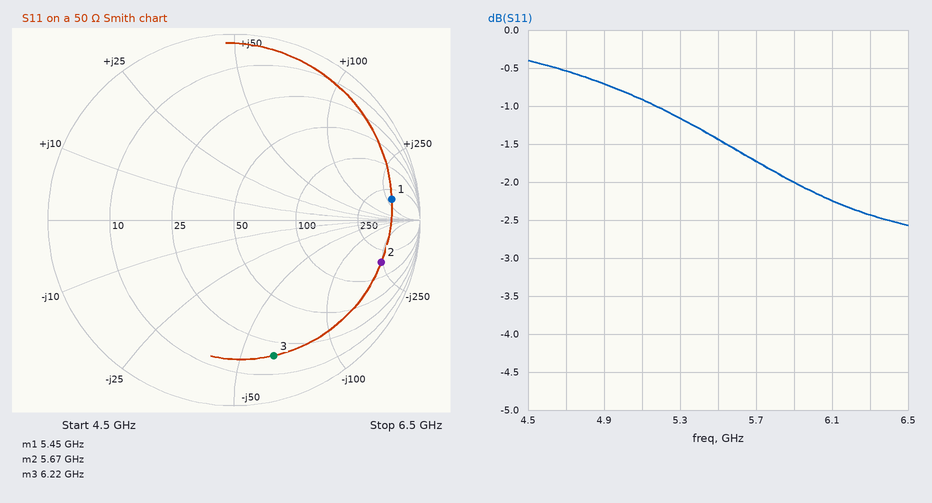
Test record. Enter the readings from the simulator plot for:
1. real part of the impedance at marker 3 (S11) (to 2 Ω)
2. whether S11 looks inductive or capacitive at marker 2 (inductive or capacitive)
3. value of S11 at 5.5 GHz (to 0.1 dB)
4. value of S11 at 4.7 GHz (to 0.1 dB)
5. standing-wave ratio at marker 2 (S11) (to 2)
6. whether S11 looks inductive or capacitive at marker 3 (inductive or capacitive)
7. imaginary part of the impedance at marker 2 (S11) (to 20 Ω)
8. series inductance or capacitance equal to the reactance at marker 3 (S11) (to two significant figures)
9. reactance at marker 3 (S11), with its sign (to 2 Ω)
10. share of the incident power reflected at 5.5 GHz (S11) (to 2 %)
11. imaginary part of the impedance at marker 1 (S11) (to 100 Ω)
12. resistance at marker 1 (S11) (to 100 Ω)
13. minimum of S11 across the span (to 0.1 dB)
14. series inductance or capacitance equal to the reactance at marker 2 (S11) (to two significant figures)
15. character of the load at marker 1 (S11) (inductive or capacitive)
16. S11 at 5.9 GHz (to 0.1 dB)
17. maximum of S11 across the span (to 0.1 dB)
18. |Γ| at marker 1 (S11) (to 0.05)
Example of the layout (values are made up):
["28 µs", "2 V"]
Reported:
["18 Ω", "capacitive", "-1.4 dB", "-0.5 dB", "10", "capacitive", "-240 Ω", "400 fF", "-64 Ω", "72 %", "+300 Ω", "400 Ω", "-2.6 dB", "120 fF", "inductive", "-2.0 dB", "-0.4 dB", "0.85"]
